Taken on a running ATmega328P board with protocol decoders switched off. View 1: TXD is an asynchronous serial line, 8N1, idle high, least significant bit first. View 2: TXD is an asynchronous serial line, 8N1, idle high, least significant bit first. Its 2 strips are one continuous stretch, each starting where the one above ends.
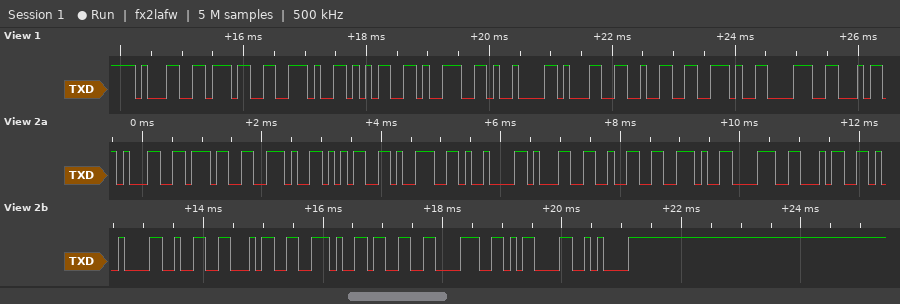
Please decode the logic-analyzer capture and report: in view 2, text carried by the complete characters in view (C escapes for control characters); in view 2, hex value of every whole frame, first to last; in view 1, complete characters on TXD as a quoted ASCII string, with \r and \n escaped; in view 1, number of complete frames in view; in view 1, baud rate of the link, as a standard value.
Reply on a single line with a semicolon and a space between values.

"17.59\t12.84\t24.38\r\n"; 31 37 2E 35 39 09 31 32 2E 38 34 09 32 34 2E 33 38 0D 0A; "17.59\t12.8"; 10; 9600 baud
